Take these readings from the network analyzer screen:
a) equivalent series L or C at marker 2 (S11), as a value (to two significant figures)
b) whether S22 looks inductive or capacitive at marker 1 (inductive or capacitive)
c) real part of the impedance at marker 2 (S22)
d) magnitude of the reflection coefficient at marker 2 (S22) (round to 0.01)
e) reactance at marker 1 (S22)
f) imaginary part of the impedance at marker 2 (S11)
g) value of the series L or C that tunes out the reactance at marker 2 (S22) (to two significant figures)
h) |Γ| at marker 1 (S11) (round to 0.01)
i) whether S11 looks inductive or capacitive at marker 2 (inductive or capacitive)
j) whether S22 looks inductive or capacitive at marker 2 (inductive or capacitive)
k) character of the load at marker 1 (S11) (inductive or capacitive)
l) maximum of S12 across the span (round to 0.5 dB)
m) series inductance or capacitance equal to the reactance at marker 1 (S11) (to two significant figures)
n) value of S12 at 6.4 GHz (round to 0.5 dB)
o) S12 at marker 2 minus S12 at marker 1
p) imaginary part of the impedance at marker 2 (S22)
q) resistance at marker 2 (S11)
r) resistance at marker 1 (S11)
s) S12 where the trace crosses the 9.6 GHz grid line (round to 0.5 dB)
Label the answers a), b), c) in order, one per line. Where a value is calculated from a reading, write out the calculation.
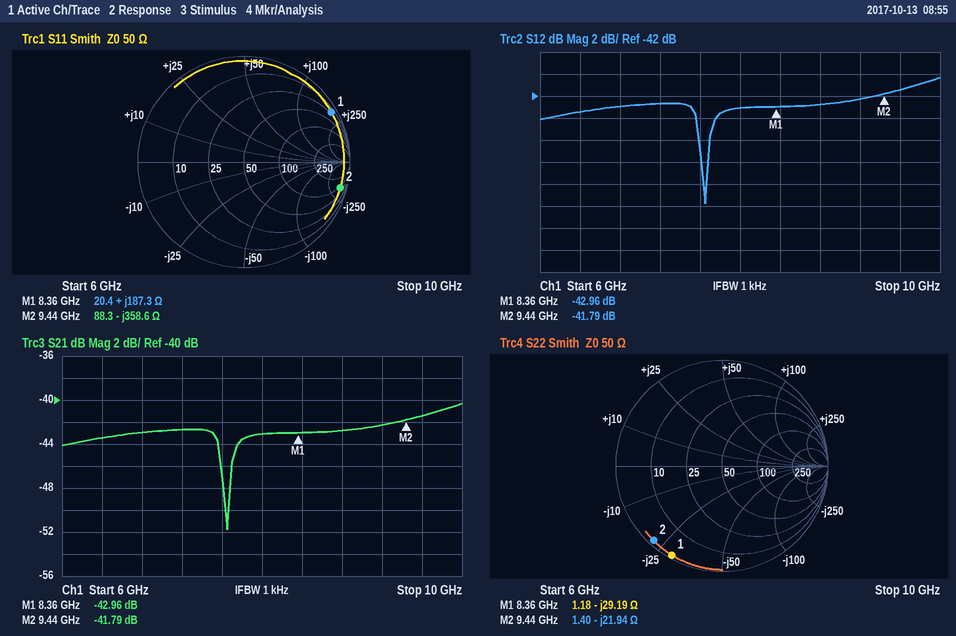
a) C = 1/(2π × 9.44 GHz × 358.6 Ω) ≈ 47 fF
b) capacitive
c) 1.40 Ω
d) 0.95
e) -29.19 Ω
f) -358.6 Ω
g) L = 21.94 Ω/(2π × 9.44 GHz) ≈ 370 pH
h) 0.95
i) capacitive
j) capacitive
k) inductive
l) -40.5 dB
m) L = 187.3 Ω/(2π × 8.36 GHz) ≈ 3.6 nH
n) -43.5 dB
o) -41.79 − (-42.96) = 1.17 dB
p) -21.94 Ω
q) 88.3 Ω
r) 20.4 Ω
s) -41.5 dB
